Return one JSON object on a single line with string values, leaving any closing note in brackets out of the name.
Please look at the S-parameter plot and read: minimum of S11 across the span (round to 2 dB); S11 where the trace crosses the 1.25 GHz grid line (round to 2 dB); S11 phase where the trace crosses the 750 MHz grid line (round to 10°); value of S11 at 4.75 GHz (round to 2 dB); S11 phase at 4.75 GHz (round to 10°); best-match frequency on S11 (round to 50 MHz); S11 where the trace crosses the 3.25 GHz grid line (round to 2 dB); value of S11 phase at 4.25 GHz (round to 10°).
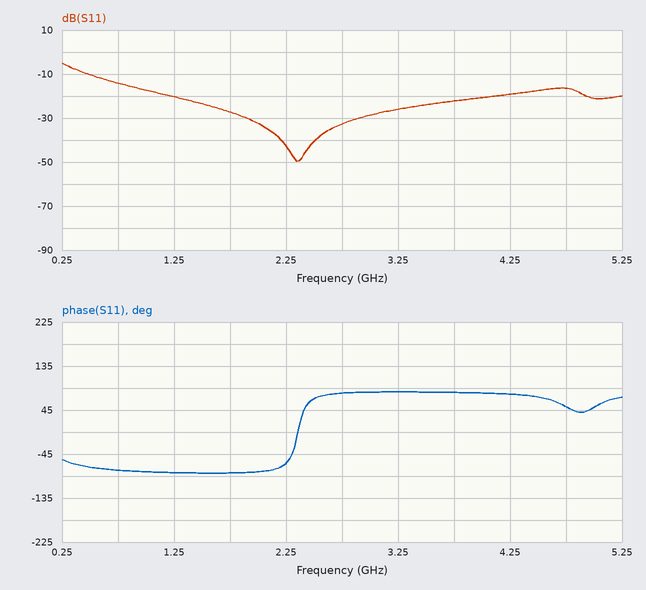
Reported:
{"minimum of S11 across the span": "-50 dB", "S11 where the trace crosses the 1.25 GHz grid line": "-20 dB", "S11 phase where the trace crosses the 750 MHz grid line": "-80°", "value of S11 at 4.75 GHz": "-16 dB", "S11 phase at 4.75 GHz": "50°", "best-match frequency on S11": "2.35 GHz", "S11 where the trace crosses the 3.25 GHz grid line": "-26 dB", "value of S11 phase at 4.25 GHz": "80°"}
